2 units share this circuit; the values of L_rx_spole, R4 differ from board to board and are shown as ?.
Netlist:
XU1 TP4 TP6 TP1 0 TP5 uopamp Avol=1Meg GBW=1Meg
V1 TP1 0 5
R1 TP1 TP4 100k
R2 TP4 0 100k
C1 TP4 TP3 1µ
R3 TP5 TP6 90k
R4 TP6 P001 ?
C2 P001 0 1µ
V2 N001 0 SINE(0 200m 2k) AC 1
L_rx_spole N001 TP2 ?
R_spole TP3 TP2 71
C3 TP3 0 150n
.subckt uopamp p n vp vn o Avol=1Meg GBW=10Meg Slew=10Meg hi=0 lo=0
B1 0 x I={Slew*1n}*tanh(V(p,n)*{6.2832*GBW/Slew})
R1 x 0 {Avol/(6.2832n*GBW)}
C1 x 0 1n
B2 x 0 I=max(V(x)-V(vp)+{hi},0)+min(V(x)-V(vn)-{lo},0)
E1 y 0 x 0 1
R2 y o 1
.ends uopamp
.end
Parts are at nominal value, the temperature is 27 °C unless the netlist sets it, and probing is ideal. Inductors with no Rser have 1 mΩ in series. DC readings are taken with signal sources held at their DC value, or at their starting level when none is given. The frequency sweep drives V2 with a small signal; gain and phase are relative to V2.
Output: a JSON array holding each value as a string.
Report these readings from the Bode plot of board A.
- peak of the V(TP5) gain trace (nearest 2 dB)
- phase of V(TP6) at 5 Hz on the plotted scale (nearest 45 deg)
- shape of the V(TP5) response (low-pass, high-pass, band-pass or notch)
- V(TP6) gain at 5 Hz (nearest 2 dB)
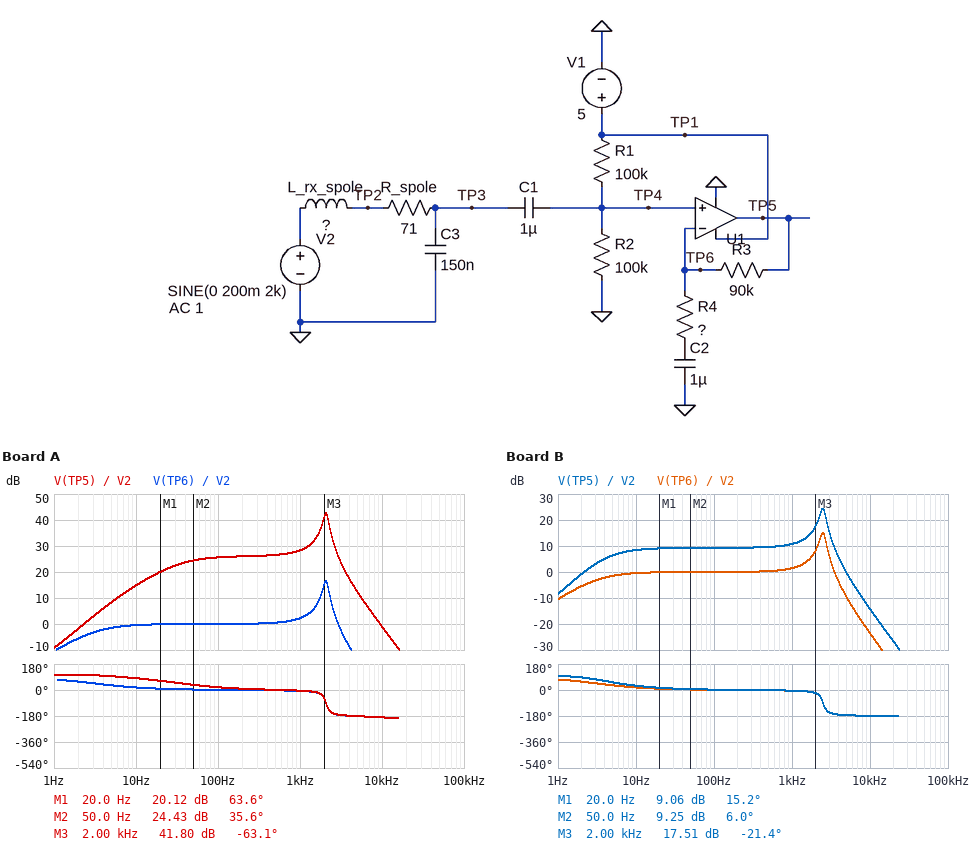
["42 dB", "45 deg", "band-pass", "-2 dB"]
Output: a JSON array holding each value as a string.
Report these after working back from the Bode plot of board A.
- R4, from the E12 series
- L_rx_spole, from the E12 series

["4.7 kΩ", "39 mH"]
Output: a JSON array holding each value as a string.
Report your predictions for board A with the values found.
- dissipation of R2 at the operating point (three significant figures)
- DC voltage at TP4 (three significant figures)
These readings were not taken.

["62.5 µW", "2.50 V"]
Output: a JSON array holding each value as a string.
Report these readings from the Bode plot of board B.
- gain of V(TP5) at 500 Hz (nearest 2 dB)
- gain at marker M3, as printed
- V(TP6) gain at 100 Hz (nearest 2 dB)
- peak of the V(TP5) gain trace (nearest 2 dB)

["10 dB", "17.51 dB", "0 dB", "24 dB"]
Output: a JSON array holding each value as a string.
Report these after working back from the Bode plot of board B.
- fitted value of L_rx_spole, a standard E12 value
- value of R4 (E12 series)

["27 mH", "47 kΩ"]
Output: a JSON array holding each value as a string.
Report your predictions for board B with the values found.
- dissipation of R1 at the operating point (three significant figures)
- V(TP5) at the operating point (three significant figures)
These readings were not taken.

["62.5 µW", "2.50 V"]
